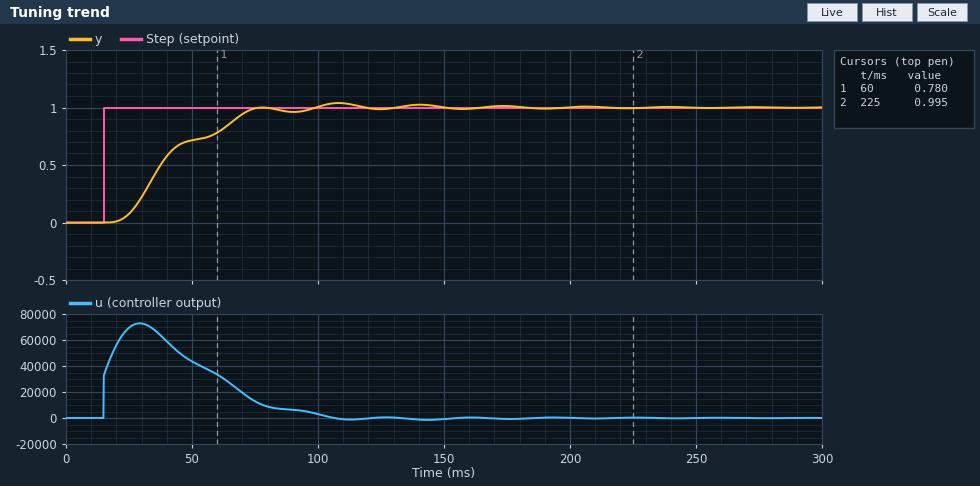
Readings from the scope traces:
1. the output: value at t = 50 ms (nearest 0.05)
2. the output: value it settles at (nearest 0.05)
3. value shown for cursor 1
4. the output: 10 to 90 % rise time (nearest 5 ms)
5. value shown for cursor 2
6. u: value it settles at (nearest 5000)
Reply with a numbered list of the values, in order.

1. 0.70
2. 1.00
3. 0.780
4. 40 ms
5. 0.995
6. 0
